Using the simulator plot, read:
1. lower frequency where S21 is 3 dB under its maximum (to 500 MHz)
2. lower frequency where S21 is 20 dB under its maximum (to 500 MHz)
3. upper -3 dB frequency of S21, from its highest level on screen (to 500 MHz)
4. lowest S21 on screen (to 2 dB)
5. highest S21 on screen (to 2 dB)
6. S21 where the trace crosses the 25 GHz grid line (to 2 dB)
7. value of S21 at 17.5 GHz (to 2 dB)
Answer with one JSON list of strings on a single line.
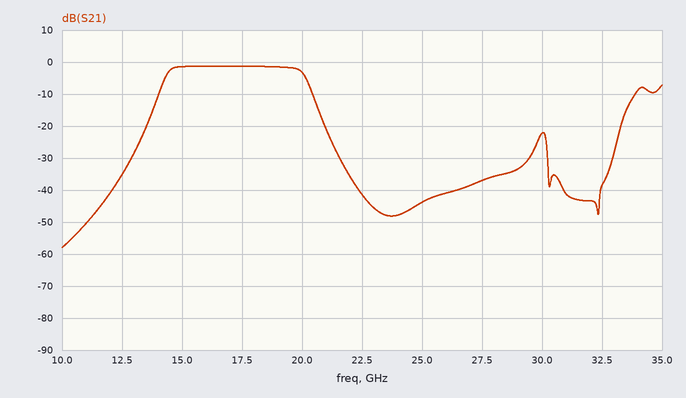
["14.5 GHz", "13.5 GHz", "20.0 GHz", "-58 dB", "-2 dB", "-44 dB", "-2 dB"]
